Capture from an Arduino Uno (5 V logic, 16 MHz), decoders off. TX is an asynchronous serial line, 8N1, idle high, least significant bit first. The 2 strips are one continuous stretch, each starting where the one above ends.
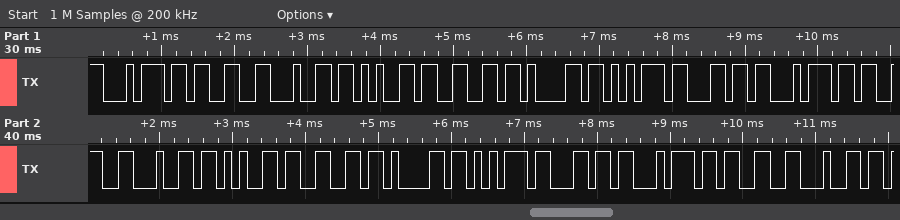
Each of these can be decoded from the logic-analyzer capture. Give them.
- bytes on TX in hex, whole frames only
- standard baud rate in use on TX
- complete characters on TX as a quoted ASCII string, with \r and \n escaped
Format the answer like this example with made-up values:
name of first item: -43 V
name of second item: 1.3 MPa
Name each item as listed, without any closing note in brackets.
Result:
bytes on TX in hex, whole frames only: 74 33 64 65 66 61 75 6C 74 33 64 65 66 61 75 6C 74 33 64
standard baud rate in use on TX: 9600 baud
complete characters on TX as a quoted ASCII string, with \r and \n escaped: "t3default3default3d"
